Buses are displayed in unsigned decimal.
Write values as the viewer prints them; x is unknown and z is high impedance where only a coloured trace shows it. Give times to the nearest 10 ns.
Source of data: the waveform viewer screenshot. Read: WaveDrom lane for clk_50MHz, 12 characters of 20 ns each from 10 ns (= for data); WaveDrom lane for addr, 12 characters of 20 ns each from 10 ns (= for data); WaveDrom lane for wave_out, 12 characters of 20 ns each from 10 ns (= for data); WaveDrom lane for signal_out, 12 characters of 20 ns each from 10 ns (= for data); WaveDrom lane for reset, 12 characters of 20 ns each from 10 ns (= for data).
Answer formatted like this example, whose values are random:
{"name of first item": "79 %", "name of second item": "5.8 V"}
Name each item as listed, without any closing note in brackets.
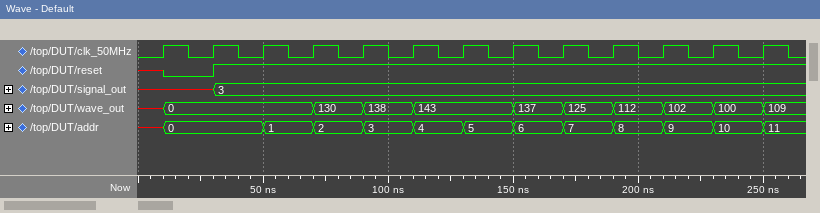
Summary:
{"WaveDrom lane for clk_50MHz, 12 characters of 20 ns each from 10 ns": "{name: 'clk_50MHz', wave: 'p...........'}", "WaveDrom lane for addr, 12 characters of 20 ns each from 10 ns": "{name: 'addr', wave: '=.==========', data: '0 1 2 3 4 5 6 7 8 9 10'}", "WaveDrom lane for wave_out, 12 characters of 20 ns each from 10 ns": "{name: 'wave_out', wave: '=..===.=====', data: '0 130 138 143 137 125 112 102 100'}", "WaveDrom lane for signal_out, 12 characters of 20 ns each from 10 ns": "{name: 'signal_out', wave: 'x=..........', data: '3'}", "WaveDrom lane for reset, 12 characters of 20 ns each from 10 ns": "{name: 'reset', wave: '01..........'}"}
